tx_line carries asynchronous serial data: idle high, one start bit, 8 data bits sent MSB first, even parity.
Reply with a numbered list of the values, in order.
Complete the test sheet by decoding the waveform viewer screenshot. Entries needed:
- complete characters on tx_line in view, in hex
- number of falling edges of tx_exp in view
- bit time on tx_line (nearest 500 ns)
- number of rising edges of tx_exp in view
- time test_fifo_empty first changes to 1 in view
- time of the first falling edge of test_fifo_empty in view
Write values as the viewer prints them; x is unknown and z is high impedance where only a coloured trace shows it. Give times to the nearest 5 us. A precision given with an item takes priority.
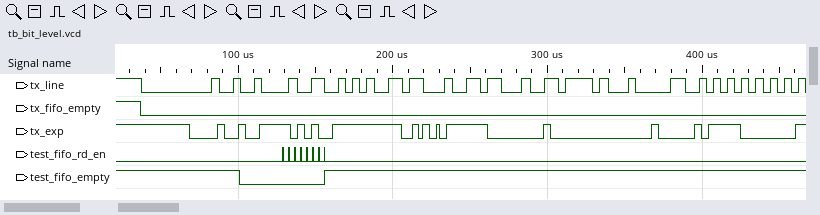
1. 00, 48, 65, 6C, 6C, 6F, 20, 55
2. 15
3. 4500 ns
4. 15
5. 155 us
6. 100 us
